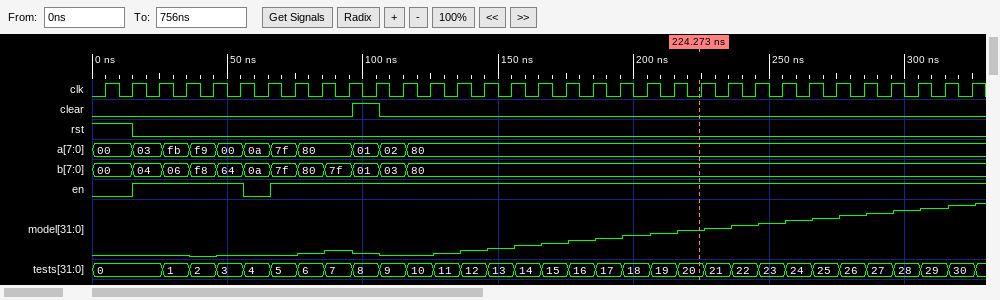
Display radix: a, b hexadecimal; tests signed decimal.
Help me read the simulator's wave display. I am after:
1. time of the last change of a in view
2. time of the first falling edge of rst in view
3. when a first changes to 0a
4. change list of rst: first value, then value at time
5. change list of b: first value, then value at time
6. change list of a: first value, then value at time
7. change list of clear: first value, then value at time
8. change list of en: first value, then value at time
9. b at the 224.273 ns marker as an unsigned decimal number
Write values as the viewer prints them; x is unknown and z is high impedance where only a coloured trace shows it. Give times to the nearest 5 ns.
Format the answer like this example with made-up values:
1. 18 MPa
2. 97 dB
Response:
1. 115 ns
2. 15 ns
3. 55 ns
4. 1, 0 at 15 ns
5. 00, 04 at 15 ns, 06 at 25 ns, f8 at 35 ns, 64 at 45 ns, 0a at 55 ns, 7f at 65 ns, 80 at 75 ns, 7f at 85 ns, 01 at 95 ns, 03 at 105 ns, 80 at 115 ns
6. 00, 03 at 15 ns, fb at 25 ns, f9 at 35 ns, 00 at 45 ns, 0a at 55 ns, 7f at 65 ns, 80 at 75 ns, 01 at 95 ns, 02 at 105 ns, 80 at 115 ns
7. 0, 1 at 95 ns, 0 at 105 ns
8. 0, 1 at 15 ns, 0 at 55 ns, 1 at 65 ns
9. 128
